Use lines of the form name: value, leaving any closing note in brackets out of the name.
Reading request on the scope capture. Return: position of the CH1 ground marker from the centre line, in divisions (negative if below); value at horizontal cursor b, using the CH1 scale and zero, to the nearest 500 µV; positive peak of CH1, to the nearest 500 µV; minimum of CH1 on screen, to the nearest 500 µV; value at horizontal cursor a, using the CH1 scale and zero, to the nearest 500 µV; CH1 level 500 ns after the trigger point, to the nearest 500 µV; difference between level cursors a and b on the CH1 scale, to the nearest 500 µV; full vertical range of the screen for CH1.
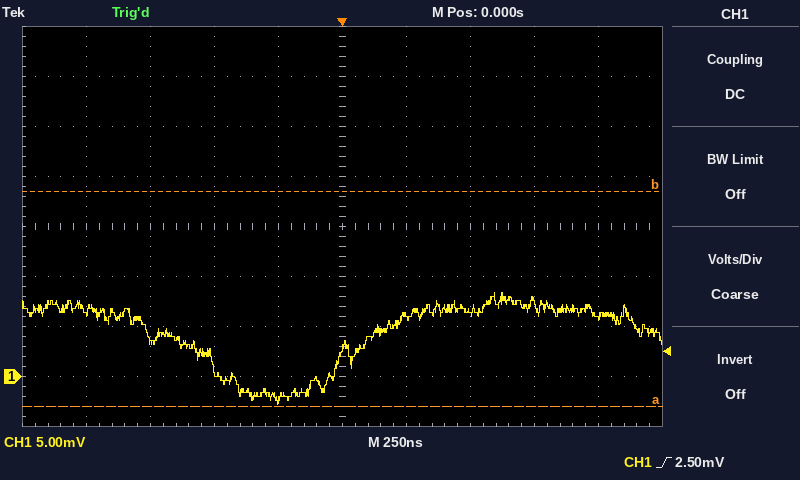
position of the CH1 ground marker from the centre line, in divisions: -3.0 div
value at horizontal cursor b, using the CH1 scale and zero, to the nearest 500 µV: 18.5 mV
positive peak of CH1, to the nearest 500 µV: 8.5 mV
minimum of CH1 on screen, to the nearest 500 µV: -3.0 mV
value at horizontal cursor a, using the CH1 scale and zero, to the nearest 500 µV: -3.0 mV
CH1 level 500 ns after the trigger point, to the nearest 500 µV: 6.5 mV
difference between level cursors a and b on the CH1 scale, to the nearest 500 µV: 21.5 mV
full vertical range of the screen for CH1: 40 mV
